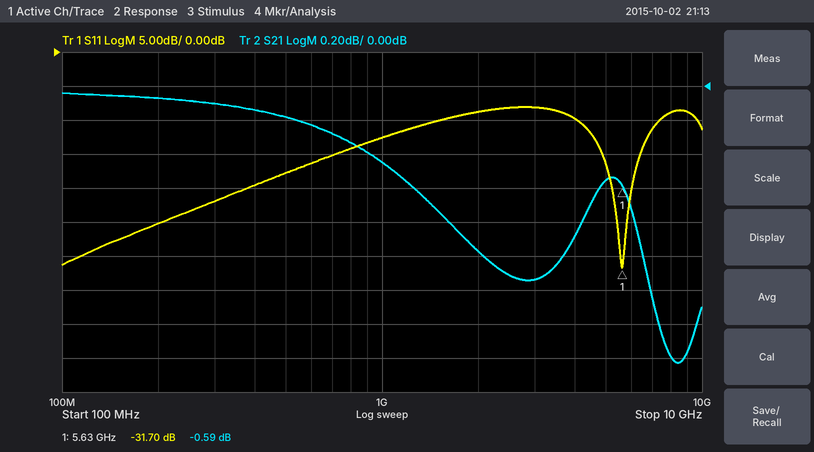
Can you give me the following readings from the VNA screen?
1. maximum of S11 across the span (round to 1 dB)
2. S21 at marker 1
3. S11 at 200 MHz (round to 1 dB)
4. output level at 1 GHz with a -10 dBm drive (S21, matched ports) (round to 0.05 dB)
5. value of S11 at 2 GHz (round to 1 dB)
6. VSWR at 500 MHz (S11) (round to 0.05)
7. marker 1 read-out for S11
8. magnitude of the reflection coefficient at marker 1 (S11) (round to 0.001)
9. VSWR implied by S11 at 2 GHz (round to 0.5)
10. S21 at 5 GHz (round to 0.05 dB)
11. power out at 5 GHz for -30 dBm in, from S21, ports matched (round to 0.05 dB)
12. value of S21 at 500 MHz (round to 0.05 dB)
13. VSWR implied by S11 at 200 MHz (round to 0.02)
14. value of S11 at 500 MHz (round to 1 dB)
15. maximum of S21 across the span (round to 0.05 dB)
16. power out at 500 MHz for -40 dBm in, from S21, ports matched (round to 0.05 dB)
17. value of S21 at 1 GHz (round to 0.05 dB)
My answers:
-8 dB
-0.59 dB
-25 dB
-10.45 dBm
-9 dB
1.30
-31.70 dB
0.026
2.0
-0.55 dB
-30.55 dBm
-0.20 dB
1.12
-18 dB
-0.05 dB
-40.20 dBm
-0.45 dB
